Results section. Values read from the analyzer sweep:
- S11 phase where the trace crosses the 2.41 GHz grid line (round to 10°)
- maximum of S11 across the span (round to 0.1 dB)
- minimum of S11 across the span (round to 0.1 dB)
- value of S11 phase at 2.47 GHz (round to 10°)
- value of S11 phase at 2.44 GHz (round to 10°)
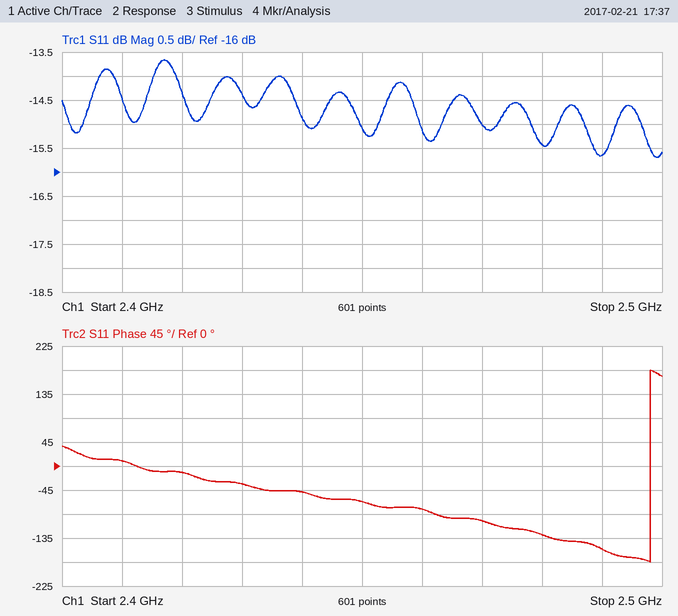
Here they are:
10°
-13.7 dB
-15.7 dB
-100°
-50°
